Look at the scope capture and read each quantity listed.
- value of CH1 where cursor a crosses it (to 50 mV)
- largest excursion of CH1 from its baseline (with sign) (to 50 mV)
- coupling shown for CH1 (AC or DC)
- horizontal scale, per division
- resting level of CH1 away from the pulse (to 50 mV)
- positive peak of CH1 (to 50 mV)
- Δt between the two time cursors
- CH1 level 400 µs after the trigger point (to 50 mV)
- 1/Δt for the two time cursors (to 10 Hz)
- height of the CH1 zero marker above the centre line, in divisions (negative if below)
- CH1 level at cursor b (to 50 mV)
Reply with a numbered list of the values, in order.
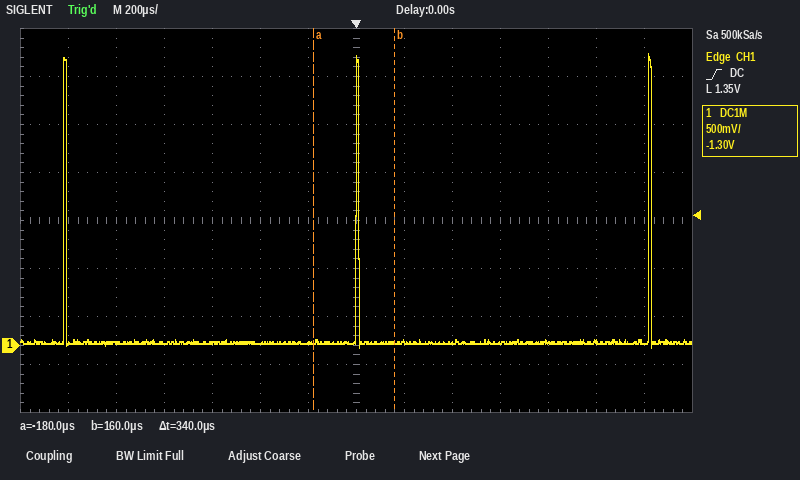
1. 50 mV
2. +3.00 V
3. DC
4. 200 µs
5. 50 mV
6. 3.05 V
7. 340 µs
8. 50 mV
9. 2.94 kHz
10. -2.6 div
11. 50 mV
